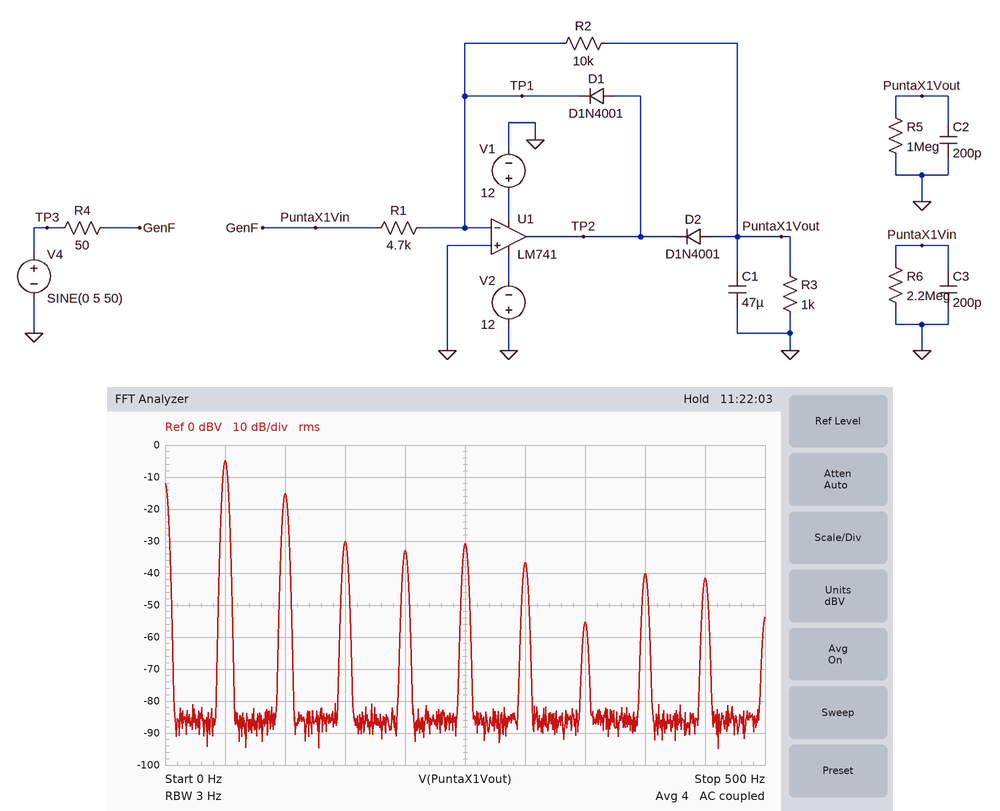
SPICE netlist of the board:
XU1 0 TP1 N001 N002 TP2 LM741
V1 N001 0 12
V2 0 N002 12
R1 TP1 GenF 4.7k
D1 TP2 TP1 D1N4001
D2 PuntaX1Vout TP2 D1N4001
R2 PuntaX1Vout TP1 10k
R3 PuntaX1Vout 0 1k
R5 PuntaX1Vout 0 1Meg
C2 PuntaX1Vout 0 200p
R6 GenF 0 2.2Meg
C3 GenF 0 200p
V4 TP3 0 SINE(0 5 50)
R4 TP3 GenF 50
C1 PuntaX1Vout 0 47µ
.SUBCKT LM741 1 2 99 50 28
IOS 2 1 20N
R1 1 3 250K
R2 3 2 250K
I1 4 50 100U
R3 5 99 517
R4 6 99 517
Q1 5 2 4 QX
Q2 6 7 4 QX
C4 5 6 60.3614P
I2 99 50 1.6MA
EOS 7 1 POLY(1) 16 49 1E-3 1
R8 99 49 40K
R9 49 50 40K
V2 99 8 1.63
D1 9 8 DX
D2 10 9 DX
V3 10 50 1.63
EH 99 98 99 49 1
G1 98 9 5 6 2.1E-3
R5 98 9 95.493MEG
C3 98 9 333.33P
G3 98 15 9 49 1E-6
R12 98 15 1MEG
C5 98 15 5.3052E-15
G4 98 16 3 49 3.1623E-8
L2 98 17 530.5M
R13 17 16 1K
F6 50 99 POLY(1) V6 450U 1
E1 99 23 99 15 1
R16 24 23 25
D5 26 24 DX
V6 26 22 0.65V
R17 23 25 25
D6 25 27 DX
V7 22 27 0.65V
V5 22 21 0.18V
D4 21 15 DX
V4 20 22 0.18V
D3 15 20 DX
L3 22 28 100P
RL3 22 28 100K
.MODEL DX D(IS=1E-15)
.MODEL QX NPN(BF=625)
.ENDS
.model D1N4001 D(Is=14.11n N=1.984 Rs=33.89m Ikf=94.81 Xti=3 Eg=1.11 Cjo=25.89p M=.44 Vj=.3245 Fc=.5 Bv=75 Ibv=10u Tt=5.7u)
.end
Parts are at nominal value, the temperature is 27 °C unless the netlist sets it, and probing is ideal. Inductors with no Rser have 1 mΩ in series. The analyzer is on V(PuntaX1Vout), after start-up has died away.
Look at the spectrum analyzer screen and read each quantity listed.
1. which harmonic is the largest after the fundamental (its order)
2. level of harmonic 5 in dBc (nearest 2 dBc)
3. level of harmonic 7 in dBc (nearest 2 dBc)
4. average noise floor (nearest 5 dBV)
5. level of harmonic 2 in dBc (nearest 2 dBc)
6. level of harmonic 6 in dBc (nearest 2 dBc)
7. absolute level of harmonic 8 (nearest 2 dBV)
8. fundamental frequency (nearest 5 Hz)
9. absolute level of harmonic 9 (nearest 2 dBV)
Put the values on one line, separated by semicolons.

2; -26 dBc; -50 dBc; -85 dBV; -10 dBc; -32 dBc; -40 dBV; 50 Hz; -42 dBV
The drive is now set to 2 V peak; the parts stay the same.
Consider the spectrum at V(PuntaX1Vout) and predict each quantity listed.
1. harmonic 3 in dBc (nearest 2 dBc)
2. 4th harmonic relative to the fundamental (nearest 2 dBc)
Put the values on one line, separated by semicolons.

-12 dBc; -18 dBc
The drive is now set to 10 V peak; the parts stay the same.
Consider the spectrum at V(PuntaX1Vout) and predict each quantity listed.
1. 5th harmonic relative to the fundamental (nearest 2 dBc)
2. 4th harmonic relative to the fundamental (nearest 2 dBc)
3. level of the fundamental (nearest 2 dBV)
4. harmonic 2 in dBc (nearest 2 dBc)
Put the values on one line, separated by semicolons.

-36 dBc; -24 dBc; -4 dBV; -14 dBc
